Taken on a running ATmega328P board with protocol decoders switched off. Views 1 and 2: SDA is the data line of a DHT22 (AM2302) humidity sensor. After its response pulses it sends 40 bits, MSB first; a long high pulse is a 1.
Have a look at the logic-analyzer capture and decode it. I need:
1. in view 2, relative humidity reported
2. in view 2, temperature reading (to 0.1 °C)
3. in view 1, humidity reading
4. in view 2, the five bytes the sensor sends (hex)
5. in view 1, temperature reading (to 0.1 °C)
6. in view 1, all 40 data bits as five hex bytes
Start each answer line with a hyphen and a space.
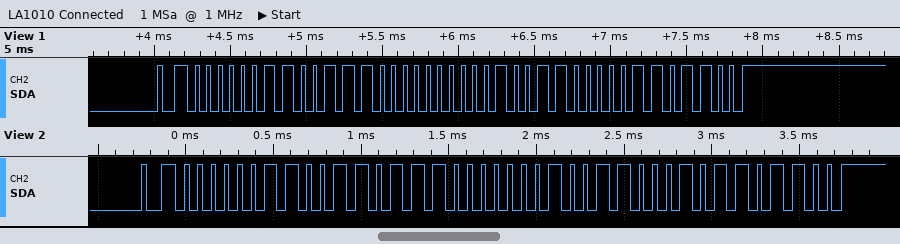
- 82.3 %
- 30.5 °C
- 82.4 %
- 03 37 01 31 6C
- 30.4 °C
- 03 38 01 30 6C
